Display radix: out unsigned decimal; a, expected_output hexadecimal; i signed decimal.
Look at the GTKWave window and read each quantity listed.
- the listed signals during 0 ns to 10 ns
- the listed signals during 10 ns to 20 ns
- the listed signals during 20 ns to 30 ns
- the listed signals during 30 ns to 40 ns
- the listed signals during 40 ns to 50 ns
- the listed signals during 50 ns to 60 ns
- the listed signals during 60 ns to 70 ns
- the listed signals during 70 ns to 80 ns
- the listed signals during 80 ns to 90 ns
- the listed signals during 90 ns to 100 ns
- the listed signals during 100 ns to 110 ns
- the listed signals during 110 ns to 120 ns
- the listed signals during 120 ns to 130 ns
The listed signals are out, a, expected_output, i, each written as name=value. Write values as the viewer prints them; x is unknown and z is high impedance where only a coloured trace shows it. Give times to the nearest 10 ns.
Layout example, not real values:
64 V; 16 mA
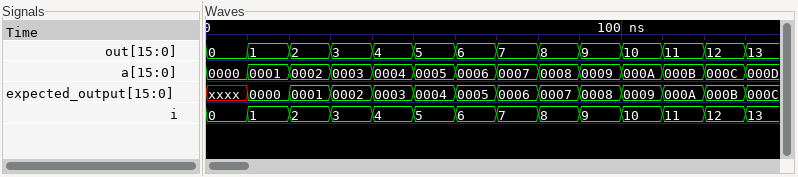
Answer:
out=0, a=0000, expected_output=xxxx, i=0; out=1, a=0001, expected_output=0000, i=1; out=2, a=0002, expected_output=0001, i=2; out=3, a=0003, expected_output=0002, i=3; out=4, a=0004, expected_output=0003, i=4; out=5, a=0005, expected_output=0004, i=5; out=6, a=0006, expected_output=0005, i=6; out=7, a=0007, expected_output=0006, i=7; out=8, a=0008, expected_output=0007, i=8; out=9, a=0009, expected_output=0008, i=9; out=10, a=000A, expected_output=0009, i=10; out=11, a=000B, expected_output=000A, i=11; out=12, a=000C, expected_output=000B, i=12
